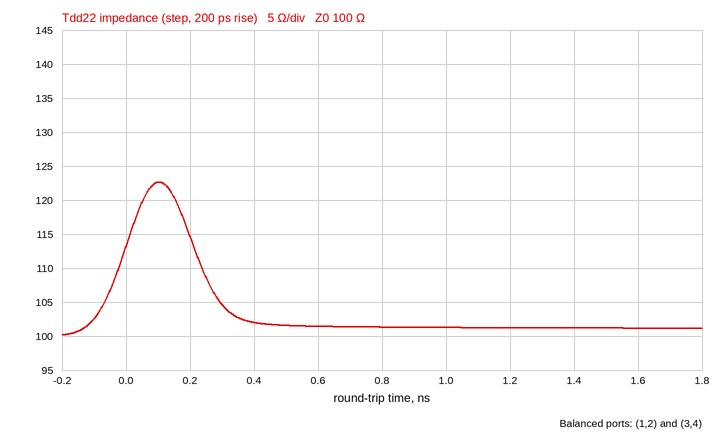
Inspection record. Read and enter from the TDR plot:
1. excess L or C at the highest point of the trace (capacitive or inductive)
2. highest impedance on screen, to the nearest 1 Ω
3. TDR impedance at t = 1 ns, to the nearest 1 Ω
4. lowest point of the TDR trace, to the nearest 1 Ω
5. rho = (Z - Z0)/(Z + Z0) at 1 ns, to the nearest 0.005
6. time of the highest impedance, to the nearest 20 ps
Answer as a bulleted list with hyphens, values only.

- inductive
- 123 Ω
- 101 Ω
- 100 Ω
- +0.005
- 100 ps
